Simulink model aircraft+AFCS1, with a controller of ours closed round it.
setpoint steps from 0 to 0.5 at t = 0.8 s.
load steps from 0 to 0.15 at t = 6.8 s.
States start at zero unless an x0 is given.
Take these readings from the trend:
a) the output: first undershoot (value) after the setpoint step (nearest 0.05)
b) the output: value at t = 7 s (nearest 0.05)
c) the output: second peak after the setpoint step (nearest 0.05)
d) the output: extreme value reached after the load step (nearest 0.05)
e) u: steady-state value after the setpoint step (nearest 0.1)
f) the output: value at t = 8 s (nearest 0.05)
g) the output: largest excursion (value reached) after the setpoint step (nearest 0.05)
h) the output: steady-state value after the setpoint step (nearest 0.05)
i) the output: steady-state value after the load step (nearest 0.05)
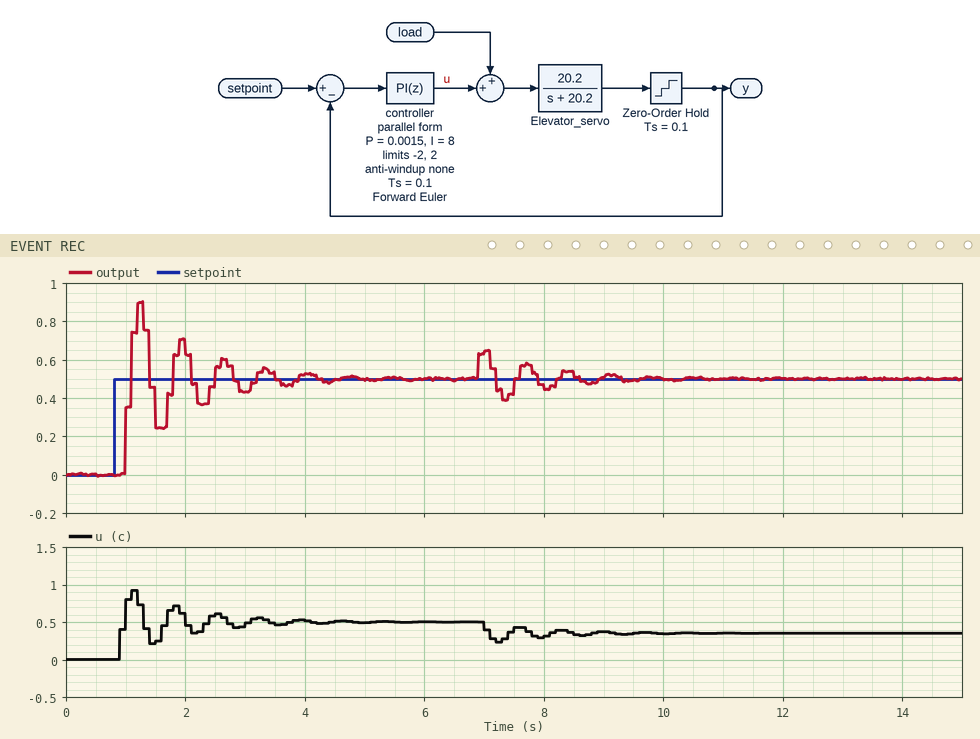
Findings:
0.25
0.65
0.70
0.65
0.5
0.45
0.90
0.50
0.50
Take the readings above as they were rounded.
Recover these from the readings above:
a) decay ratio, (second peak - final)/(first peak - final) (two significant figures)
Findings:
0.50
